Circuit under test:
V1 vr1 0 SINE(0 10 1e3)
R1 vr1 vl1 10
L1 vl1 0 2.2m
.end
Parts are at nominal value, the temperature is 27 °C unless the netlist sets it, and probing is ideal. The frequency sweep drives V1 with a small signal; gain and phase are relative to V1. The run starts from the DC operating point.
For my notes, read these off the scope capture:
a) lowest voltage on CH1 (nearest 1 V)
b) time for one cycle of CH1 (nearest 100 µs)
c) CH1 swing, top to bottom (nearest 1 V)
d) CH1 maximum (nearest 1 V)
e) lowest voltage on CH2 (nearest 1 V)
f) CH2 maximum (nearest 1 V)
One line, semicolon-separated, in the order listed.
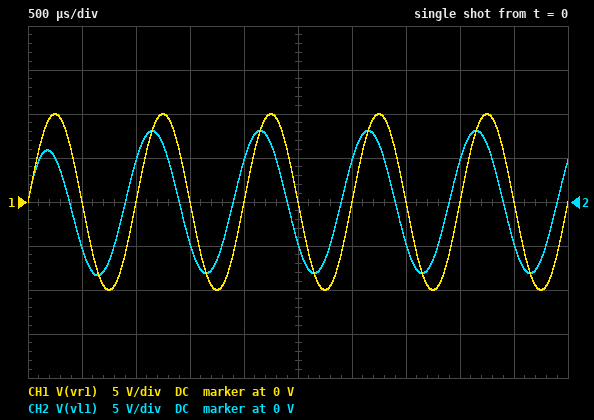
-10 V; 1.0 ms; 20 V; 10 V; -8 V; 8 V
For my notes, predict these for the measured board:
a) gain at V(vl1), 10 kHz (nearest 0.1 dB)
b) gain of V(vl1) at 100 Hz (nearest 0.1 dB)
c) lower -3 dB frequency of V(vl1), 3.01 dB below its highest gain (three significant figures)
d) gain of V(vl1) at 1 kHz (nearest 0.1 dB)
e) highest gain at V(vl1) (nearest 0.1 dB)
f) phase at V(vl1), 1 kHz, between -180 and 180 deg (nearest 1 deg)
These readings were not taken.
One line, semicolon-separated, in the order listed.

0 dB; -17.3 dB; 723 Hz; -1.8 dB; 0 dB; 36 deg
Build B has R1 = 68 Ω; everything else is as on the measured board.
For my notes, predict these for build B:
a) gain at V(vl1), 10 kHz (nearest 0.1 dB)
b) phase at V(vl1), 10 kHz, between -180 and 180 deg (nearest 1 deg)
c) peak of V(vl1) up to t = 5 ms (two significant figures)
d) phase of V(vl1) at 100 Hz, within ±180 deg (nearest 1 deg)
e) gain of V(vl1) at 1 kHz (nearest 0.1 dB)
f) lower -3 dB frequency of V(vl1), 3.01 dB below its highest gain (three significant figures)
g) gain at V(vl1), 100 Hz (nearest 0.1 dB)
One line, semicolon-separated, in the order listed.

-0.9 dB; 26 deg; 2.0 V; 89 deg; -14.0 dB; 4.92 kHz; -33.8 dB
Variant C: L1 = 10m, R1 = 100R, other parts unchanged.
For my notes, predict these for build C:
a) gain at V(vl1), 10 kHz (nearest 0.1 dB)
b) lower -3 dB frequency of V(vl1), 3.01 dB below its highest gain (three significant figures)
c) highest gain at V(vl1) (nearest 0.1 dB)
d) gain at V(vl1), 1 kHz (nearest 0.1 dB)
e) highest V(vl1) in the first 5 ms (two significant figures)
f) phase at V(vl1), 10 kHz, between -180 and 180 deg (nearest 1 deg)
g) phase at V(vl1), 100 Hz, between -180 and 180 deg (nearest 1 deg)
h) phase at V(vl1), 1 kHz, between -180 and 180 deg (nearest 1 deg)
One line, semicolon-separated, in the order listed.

-0.1 dB; 1.59 kHz; 0 dB; -5.5 dB; 5.3 V; 9 deg; 86 deg; 58 deg
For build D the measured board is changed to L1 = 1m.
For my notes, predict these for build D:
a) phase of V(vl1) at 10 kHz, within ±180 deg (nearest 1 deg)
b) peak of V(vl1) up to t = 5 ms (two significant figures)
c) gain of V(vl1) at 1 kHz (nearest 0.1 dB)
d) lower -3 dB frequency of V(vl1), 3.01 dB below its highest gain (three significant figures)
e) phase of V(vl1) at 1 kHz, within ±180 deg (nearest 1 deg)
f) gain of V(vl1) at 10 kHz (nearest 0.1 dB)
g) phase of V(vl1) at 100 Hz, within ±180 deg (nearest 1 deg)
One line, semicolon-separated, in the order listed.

9 deg; 5.3 V; -5.5 dB; 1.59 kHz; 58 deg; -0.1 dB; 86 deg
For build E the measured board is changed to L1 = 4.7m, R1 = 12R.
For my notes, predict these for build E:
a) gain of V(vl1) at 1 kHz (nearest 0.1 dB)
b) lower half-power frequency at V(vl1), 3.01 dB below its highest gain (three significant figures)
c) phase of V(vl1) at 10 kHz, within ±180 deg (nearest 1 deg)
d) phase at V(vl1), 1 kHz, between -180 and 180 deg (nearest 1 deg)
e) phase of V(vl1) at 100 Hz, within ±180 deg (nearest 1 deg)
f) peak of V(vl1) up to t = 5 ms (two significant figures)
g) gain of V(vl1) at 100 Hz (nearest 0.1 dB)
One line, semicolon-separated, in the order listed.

-0.7 dB; 406 Hz; 2 deg; 22 deg; 76 deg; 9.3 V; -12.4 dB
